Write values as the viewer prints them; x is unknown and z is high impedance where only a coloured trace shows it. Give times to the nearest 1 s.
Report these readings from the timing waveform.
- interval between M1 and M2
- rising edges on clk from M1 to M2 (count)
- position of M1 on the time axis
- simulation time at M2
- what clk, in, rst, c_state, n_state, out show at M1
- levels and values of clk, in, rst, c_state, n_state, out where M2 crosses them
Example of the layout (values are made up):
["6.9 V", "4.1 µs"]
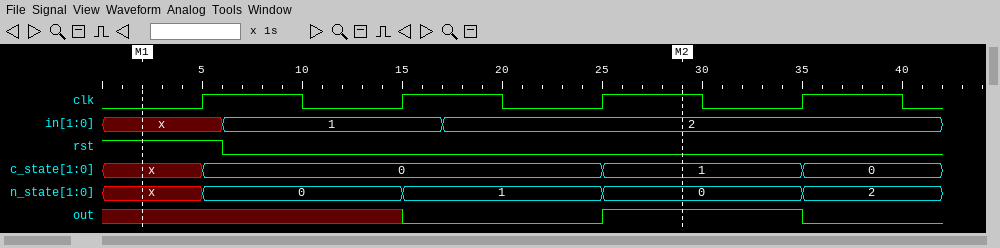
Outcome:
["27 s", "3", "2 s", "29 s", "clk=0, in=x, rst=1, c_state=x, n_state=x, out=x", "clk=1, in=2, rst=0, c_state=1, n_state=0, out=1"]
